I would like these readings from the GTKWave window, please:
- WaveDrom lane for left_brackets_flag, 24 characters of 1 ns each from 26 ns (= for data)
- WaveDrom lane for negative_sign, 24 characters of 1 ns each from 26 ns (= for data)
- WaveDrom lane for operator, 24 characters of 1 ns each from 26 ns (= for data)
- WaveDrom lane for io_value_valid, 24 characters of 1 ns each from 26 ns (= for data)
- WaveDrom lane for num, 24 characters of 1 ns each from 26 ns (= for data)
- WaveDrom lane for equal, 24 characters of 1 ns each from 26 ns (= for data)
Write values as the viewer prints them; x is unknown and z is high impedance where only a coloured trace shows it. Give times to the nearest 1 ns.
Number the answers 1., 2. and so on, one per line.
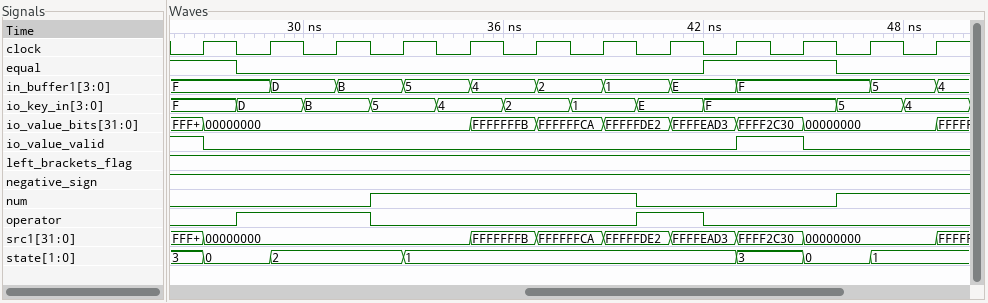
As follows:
1. {name: 'left_brackets_flag', wave: '1.......................'}
2. {name: 'negative_sign', wave: '1.......................'}
3. {name: 'operator', wave: '0.1...0.......1.0.......'}
4. {name: 'io_value_valid', wave: '10...............1.0....'}
5. {name: 'num', wave: '0.....1.......0.....1...'}
6. {name: 'equal', wave: '1.0.............1...0...'}
